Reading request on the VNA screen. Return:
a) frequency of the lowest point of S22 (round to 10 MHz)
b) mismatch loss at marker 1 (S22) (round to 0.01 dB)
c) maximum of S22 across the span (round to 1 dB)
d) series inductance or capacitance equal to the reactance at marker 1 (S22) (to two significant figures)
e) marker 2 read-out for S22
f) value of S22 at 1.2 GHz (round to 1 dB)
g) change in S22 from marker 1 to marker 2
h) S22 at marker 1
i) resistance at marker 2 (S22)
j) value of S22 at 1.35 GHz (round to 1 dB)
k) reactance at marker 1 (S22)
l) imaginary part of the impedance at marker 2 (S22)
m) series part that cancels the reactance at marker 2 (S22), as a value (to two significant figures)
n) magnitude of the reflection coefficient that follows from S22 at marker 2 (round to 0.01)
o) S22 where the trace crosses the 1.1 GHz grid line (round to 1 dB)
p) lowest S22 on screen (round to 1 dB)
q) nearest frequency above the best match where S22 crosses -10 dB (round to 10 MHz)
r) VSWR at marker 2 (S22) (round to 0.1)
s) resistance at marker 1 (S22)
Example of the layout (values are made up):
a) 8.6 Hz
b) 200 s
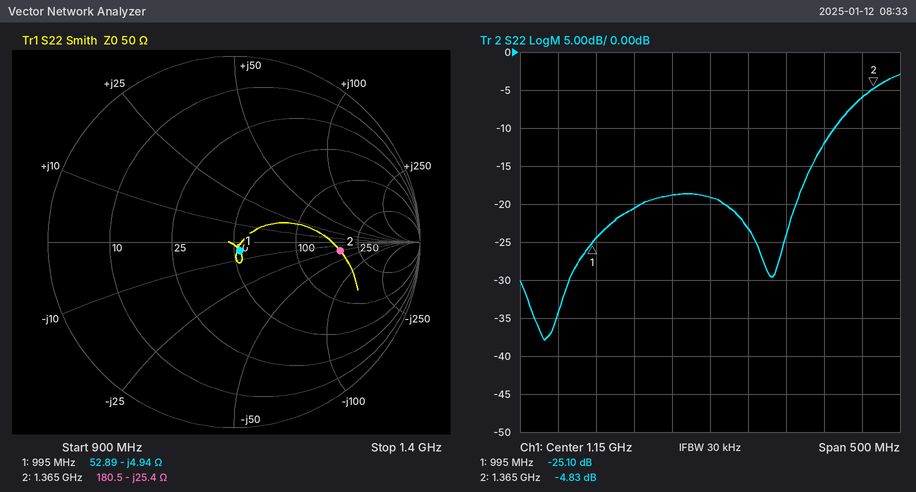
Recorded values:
a) 930 MHz
b) 0.01 dB
c) -3 dB
d) 32 pF
e) -4.83 dB
f) -23 dB
g) 20.27 dB
h) -25.10 dB
i) 180.5 Ω
j) -6 dB
k) -4.94 Ω
l) -25.4 Ω
m) 3.0 nH
n) 0.57
o) -19 dB
p) -38 dB
q) 1.31 GHz
r) 3.7
s) 52.89 Ω
